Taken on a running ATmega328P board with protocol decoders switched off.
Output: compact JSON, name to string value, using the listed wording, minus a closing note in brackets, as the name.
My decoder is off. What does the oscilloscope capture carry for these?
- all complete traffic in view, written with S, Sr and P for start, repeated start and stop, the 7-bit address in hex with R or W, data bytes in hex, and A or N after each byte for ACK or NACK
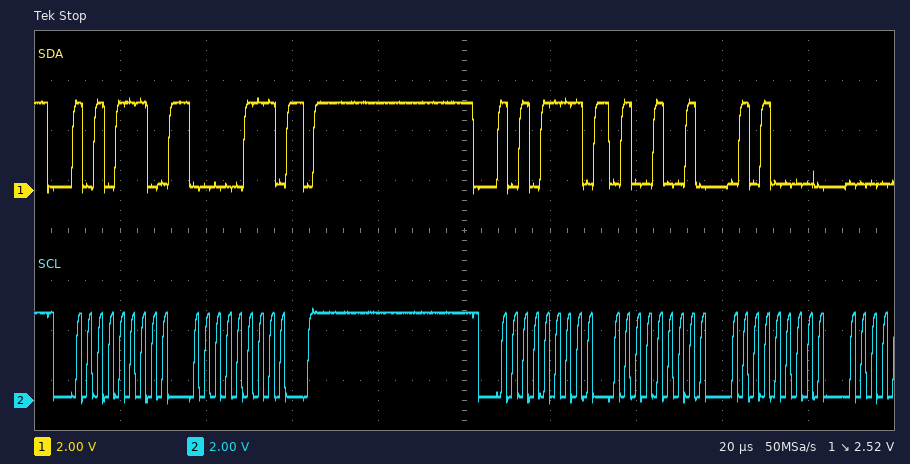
{"all complete traffic in view, written with S, Sr and P for start, repeated start and stop, the 7-bit address in hex with R or W, data bytes in hex, and A or N after each byte for ACK or NACK": "S 57W A 07 A P S 57R A 49 A 50 A"}
